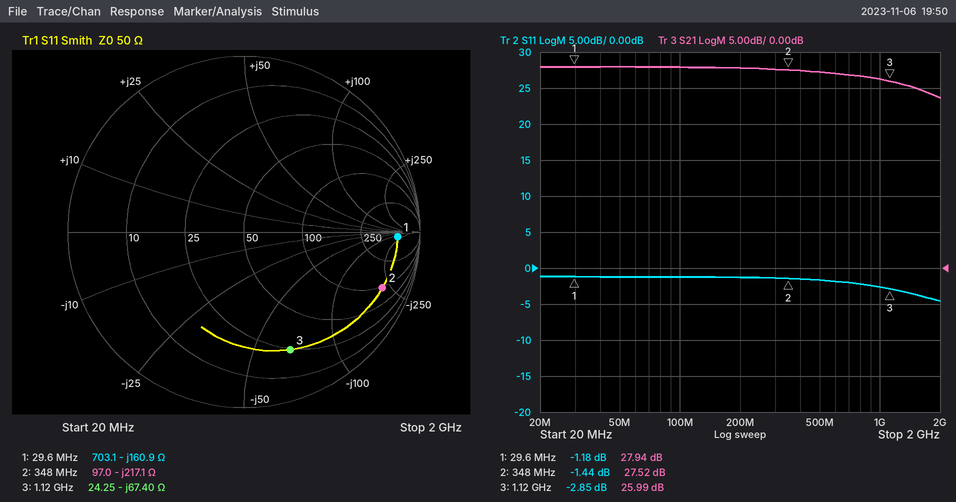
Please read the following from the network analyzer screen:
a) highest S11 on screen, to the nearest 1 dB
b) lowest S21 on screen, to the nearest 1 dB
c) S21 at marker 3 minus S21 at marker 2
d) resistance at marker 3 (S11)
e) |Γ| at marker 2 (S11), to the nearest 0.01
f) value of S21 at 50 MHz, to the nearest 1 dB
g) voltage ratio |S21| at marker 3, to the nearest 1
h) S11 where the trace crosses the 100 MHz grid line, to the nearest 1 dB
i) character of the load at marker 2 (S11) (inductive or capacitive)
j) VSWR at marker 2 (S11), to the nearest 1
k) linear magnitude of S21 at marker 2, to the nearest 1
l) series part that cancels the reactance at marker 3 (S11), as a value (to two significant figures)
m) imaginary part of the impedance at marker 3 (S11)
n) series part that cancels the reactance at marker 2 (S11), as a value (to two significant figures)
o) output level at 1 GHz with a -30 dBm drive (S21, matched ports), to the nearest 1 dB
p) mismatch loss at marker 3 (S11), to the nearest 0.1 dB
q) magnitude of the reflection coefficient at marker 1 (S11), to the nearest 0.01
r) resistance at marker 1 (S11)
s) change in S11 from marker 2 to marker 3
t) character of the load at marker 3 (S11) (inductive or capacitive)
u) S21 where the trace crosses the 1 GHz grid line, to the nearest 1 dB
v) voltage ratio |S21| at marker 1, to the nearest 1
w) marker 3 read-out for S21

-1 dB
24 dB
-1.53 dB
24.25 Ω
0.85
28 dB
20
-1 dB
capacitive
12
24
9.6 nH
-67.40 Ω
99 nH
-4 dBm
3.2 dB
0.87
703.1 Ω
-1.41 dB
capacitive
26 dB
25
25.99 dB
